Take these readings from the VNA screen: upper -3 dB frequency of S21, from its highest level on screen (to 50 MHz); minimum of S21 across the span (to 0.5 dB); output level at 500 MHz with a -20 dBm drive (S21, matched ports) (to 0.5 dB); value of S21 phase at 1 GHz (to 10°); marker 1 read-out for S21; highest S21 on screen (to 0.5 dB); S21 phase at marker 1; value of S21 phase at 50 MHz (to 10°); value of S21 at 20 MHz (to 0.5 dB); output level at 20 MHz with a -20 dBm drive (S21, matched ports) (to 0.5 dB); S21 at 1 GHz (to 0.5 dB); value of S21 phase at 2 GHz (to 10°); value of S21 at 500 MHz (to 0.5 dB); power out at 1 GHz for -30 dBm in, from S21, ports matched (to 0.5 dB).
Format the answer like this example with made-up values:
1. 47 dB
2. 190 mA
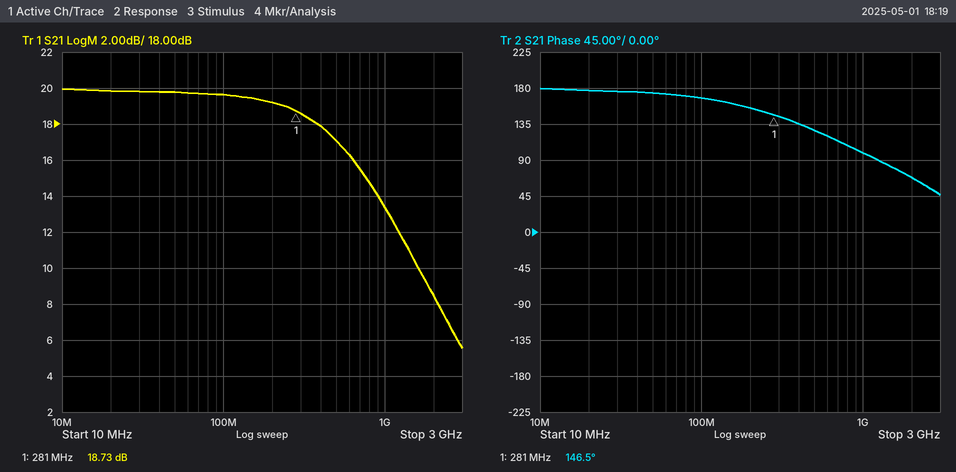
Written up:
1. 500 MHz
2. 5.5 dB
3. -3.0 dBm
4. 100°
5. 18.73 dB
6. 20.0 dB
7. 146.5°
8. 170°
9. 20.0 dB
10. 0.0 dBm
11. 13.5 dB
12. 70°
13. 17.0 dB
14. -16.5 dBm
